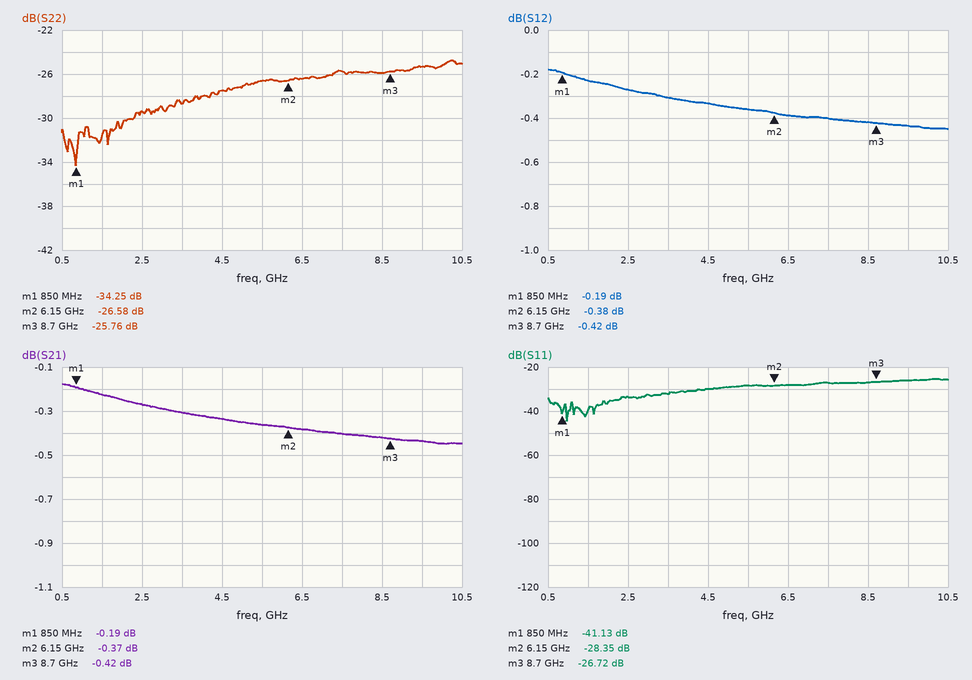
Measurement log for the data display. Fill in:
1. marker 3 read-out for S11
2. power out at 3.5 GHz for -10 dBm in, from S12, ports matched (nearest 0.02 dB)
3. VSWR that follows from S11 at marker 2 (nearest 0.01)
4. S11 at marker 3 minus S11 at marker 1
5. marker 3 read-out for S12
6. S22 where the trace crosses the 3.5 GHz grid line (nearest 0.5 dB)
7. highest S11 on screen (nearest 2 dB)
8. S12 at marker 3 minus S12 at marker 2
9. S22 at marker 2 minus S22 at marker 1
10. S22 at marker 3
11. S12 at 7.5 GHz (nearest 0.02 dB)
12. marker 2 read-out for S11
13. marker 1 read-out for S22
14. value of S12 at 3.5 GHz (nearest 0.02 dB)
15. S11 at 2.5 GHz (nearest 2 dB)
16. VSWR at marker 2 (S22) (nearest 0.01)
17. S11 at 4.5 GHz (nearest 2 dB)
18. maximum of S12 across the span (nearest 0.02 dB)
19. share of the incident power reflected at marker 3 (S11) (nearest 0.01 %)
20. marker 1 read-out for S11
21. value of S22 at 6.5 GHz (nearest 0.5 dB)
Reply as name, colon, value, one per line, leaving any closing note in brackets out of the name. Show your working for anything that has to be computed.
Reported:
marker 3 read-out for S11: -26.72 dB
power out at 3.5 GHz for -10 dBm in, from S12, ports matched: -10 dBm + (-0.30 dB) = -10.30 dBm
VSWR that follows from S11 at marker 2: (1 + 0.0382)/(1 − 0.0382) ≈ 1.08
S11 at marker 3 minus S11 at marker 1: -26.72 − (-41.13) = 14.41 dB
marker 3 read-out for S12: -0.42 dB
S22 where the trace crosses the 3.5 GHz grid line: -28.5 dB
highest S11 on screen: -26 dB
S12 at marker 3 minus S12 at marker 2: -0.42 − (-0.38) = -0.04 dB
S22 at marker 2 minus S22 at marker 1: -26.58 − (-34.25) = 7.67 dB
S22 at marker 3: -25.76 dB
S12 at 7.5 GHz: -0.40 dB
marker 2 read-out for S11: -28.35 dB
marker 1 read-out for S22: -34.25 dB
value of S12 at 3.5 GHz: -0.30 dB
S11 at 2.5 GHz: -34 dB
VSWR at marker 2 (S22): (1 + 0.0469)/(1 − 0.0469) ≈ 1.10
S11 at 4.5 GHz: -30 dB
maximum of S12 across the span: -0.18 dB
share of the incident power reflected at marker 3 (S11): 10^(-26.72/10) ≈ 0.21 %
marker 1 read-out for S11: -41.13 dB
value of S22 at 6.5 GHz: -26.5 dB
